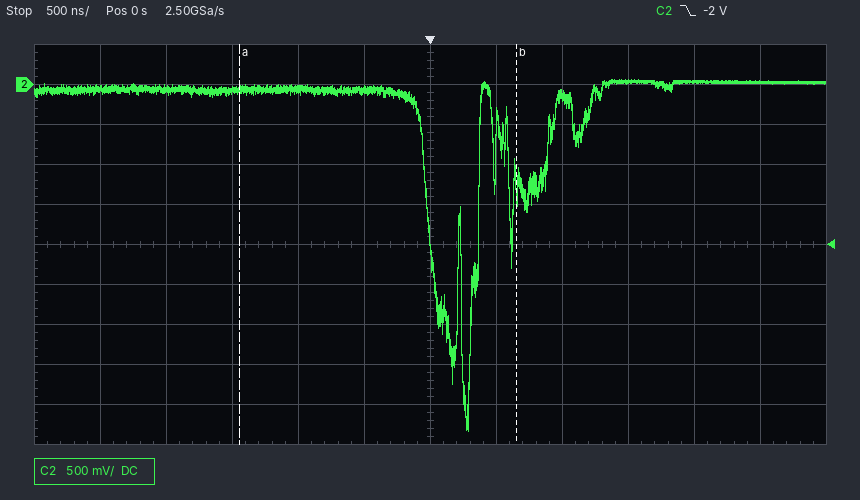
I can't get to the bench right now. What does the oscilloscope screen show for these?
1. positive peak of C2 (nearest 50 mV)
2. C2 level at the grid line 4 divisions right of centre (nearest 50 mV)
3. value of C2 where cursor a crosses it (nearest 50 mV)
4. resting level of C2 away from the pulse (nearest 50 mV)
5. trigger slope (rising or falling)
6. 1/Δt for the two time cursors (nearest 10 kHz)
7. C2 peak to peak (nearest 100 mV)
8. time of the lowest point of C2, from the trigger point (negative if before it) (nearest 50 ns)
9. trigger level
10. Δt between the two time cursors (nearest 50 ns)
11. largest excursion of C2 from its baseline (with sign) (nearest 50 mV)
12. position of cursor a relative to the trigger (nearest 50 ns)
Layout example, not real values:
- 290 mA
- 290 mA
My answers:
- 50 mV
- 50 mV
- -50 mV
- -50 mV
- falling
- 480 kHz
- 4.40 V
- +300 ns
- -2 V
- 2.10 µs
- -4.25 V
- -1.45 µs
